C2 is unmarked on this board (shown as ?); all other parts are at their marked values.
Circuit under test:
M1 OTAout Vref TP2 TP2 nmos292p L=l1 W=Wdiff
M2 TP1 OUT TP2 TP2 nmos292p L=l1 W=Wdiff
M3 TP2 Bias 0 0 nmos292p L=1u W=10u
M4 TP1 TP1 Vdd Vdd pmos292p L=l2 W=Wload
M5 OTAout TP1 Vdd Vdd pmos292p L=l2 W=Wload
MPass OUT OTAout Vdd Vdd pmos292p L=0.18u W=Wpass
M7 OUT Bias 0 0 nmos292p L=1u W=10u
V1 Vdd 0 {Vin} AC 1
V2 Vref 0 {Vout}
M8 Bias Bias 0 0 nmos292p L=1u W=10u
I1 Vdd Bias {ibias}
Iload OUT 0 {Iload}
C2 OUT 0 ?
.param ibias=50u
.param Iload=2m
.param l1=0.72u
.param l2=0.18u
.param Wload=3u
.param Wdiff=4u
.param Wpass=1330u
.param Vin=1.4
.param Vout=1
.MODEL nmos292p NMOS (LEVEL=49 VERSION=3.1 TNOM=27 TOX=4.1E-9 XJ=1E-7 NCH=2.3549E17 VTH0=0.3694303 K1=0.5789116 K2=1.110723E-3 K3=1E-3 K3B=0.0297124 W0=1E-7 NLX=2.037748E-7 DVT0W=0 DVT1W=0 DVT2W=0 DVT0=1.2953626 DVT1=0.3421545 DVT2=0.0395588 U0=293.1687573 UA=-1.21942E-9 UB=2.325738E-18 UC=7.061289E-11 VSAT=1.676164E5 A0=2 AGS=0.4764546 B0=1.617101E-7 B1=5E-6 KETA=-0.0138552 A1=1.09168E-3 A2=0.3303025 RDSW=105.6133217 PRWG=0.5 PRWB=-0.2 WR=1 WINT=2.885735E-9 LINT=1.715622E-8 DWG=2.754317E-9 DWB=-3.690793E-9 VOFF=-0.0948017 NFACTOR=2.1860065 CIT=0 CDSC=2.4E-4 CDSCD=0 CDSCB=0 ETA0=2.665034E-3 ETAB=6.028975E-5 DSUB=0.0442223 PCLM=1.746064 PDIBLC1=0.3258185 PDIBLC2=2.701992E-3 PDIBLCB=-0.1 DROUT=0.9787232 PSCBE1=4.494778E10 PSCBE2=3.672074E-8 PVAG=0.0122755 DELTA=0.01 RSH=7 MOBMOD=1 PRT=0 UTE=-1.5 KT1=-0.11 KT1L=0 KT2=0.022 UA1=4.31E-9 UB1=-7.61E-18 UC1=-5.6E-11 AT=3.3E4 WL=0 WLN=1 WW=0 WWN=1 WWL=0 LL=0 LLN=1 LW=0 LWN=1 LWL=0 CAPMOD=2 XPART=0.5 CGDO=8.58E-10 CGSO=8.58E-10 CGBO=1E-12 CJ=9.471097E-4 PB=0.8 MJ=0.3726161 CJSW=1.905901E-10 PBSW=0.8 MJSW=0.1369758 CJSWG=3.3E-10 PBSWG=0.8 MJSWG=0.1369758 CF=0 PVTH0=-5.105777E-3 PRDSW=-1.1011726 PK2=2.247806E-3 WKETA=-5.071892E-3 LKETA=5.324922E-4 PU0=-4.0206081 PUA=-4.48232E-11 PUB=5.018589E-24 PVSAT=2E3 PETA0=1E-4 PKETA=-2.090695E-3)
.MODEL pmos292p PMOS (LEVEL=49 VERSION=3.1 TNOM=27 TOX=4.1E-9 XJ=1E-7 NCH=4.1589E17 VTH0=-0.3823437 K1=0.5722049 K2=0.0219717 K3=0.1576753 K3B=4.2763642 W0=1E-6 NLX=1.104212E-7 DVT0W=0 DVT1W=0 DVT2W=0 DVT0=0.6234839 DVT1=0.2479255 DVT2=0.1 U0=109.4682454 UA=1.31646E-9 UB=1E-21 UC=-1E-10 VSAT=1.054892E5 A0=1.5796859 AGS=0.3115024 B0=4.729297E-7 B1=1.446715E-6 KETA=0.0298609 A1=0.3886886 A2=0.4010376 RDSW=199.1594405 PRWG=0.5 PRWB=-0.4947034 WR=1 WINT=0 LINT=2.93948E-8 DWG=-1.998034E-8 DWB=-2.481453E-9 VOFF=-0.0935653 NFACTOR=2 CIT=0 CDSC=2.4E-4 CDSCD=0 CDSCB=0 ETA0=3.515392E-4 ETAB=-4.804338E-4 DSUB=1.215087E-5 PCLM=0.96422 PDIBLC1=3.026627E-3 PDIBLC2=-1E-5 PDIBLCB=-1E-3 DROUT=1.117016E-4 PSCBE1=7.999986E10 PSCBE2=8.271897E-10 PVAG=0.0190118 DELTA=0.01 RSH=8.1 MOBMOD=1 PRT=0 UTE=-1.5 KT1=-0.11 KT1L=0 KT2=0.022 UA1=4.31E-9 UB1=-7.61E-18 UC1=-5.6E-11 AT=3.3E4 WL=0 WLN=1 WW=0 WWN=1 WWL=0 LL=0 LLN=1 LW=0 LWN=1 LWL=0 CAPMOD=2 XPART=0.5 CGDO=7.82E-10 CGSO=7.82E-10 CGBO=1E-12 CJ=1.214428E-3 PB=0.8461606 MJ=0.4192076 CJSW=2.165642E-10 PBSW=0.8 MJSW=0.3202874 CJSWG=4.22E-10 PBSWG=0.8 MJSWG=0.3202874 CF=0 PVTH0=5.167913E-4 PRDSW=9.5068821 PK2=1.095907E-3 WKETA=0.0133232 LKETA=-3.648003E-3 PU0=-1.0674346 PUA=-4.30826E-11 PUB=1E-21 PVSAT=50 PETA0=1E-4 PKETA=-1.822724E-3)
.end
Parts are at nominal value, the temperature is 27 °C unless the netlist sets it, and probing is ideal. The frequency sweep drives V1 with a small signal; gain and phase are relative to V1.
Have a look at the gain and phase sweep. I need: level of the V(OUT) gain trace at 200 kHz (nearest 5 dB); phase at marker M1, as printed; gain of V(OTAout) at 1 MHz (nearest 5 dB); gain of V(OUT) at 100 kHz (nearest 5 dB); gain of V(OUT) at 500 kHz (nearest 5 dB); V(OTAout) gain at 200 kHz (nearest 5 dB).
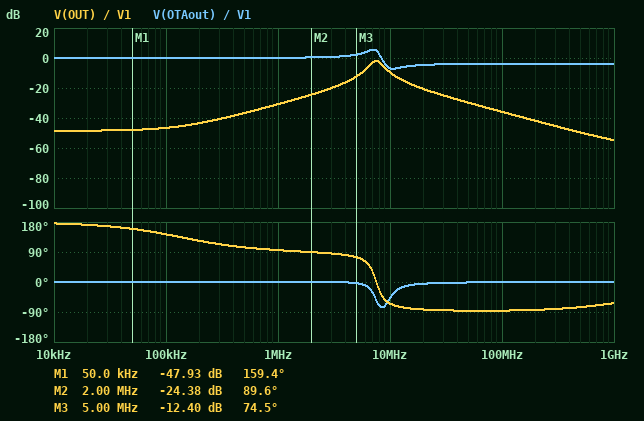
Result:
-45 dB
159.4 deg
0 dB
-45 dB
-35 dB
0 dB
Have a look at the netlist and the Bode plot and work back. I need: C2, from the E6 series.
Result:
1 nF
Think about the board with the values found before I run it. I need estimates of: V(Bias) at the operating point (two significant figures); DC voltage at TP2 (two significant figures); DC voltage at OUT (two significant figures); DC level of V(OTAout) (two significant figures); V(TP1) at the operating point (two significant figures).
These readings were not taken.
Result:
620 mV
380 mV
1.0 V
840 mV
750 mV
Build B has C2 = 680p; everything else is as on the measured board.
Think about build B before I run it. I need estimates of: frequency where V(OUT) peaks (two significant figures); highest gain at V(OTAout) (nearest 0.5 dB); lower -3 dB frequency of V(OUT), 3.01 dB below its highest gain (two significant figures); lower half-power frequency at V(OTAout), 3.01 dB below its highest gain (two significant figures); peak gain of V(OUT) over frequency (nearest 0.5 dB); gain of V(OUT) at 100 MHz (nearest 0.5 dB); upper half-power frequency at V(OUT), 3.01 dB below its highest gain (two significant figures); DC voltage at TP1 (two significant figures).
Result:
9.1 MHz
5.0 dB
7.9 MHz
5.8 MHz
-1.0 dB
-32.5 dB
11 MHz
750 mV
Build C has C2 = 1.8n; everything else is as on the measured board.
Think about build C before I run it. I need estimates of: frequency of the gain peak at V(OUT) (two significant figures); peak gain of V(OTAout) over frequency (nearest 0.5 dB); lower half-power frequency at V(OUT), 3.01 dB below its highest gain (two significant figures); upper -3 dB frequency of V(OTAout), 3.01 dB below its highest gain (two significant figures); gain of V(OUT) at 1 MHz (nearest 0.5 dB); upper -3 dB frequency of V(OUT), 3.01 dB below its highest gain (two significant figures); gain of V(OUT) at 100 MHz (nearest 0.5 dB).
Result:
5.6 MHz
6.5 dB
5.0 MHz
5.9 MHz
-30.5 dB
6.3 MHz
-41.0 dB
